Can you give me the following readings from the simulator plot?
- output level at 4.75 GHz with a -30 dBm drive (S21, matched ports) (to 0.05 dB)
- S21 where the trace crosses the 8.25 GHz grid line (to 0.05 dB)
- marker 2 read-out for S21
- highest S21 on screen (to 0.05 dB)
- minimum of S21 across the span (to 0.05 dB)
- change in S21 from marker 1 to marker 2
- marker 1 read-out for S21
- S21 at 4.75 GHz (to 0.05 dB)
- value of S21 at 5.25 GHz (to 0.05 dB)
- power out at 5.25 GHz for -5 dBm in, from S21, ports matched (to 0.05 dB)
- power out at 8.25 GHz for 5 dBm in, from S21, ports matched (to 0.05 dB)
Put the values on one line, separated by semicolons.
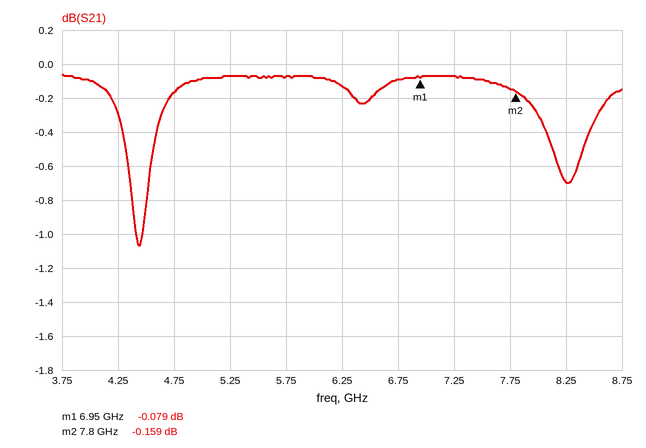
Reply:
-30.15 dBm; -0.70 dB; -0.159 dB; -0.05 dB; -1.05 dB; -0.080 dB; -0.079 dB; -0.15 dB; -0.05 dB; -5.05 dBm; 4.30 dBm
